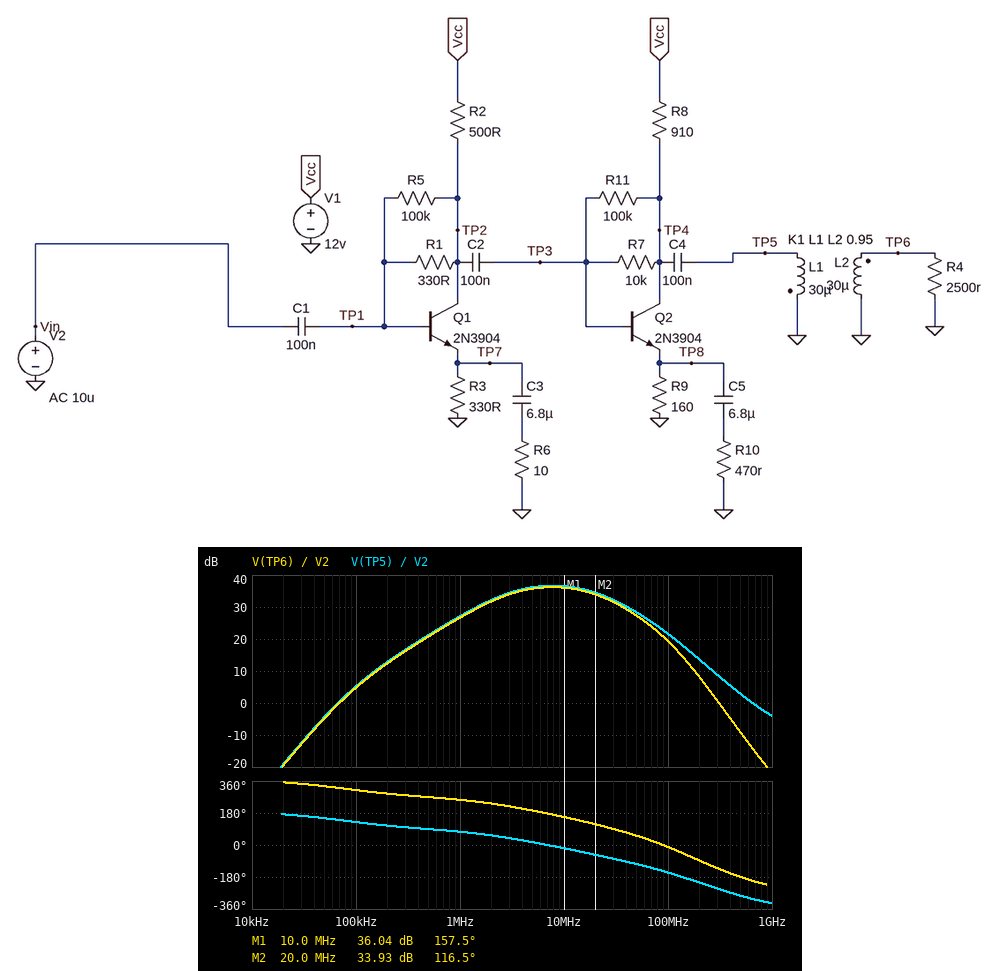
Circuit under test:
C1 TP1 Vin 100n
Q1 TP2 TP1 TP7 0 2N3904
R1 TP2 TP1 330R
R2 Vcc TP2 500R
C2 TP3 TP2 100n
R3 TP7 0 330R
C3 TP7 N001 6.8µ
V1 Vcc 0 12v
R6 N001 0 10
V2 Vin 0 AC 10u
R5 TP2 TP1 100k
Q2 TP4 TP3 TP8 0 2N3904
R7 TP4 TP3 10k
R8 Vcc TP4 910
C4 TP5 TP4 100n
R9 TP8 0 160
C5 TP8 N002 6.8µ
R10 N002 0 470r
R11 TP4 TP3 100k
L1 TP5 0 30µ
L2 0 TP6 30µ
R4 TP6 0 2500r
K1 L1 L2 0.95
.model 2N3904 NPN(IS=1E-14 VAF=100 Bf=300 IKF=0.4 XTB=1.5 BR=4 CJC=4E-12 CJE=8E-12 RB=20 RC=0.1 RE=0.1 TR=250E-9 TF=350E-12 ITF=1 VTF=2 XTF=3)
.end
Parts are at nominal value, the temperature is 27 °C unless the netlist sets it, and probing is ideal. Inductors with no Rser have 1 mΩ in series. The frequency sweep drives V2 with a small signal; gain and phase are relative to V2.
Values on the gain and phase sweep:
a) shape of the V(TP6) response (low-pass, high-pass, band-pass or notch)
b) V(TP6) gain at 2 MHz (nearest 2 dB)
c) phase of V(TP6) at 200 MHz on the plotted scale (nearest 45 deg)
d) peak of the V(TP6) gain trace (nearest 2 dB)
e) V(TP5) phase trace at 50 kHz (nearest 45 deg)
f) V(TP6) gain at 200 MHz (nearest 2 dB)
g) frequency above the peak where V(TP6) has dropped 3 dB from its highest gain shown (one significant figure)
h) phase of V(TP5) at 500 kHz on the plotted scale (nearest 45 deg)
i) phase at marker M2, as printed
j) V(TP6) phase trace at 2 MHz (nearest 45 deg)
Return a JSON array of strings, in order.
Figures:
["band-pass", "32 dB", "-90 deg", "36 dB", "135 deg", "8 dB", "20 MHz", "90 deg", "116.5 deg", "225 deg"]
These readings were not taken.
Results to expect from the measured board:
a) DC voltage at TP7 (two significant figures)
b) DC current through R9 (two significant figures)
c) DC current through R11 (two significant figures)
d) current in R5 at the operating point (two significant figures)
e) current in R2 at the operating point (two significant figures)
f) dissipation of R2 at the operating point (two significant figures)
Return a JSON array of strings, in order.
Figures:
["4.5 V", "10 mA", "3.2 µA", "150 nA", "14 mA", "92 mW"]
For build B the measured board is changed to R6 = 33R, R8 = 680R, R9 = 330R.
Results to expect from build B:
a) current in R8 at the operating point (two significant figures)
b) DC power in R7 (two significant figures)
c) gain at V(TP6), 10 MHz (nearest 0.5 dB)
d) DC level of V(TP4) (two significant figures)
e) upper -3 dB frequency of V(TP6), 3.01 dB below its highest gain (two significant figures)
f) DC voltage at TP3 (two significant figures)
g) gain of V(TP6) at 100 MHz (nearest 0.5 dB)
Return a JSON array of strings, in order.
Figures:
["11 mA", "11 µW", "21.5 dB", "4.6 V", "33 MHz", "4.3 V", "10.0 dB"]
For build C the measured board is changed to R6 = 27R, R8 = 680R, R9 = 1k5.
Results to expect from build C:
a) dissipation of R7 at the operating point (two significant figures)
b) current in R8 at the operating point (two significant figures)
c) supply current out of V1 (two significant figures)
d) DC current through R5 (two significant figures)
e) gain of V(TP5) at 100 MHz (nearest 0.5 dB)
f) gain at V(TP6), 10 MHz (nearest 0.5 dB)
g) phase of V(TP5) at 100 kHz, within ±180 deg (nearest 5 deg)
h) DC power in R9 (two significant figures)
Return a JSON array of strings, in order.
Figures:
["2.4 µW", "5.1 mA", "19 mA", "150 nA", "11.5 dB", "18.0 dB", "110 deg", "39 mW"]
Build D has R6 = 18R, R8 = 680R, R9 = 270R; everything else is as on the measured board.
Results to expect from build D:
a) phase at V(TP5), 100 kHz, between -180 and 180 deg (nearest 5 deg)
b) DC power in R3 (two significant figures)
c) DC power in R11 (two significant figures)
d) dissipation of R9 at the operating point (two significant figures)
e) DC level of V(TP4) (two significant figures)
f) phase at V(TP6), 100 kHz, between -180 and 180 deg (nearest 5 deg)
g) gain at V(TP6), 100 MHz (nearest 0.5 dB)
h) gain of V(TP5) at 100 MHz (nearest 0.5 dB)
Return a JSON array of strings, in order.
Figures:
["115 deg", "61 mW", "1.3 µW", "36 mW", "4.2 V", "-65 deg", "14.5 dB", "16.5 dB"]
